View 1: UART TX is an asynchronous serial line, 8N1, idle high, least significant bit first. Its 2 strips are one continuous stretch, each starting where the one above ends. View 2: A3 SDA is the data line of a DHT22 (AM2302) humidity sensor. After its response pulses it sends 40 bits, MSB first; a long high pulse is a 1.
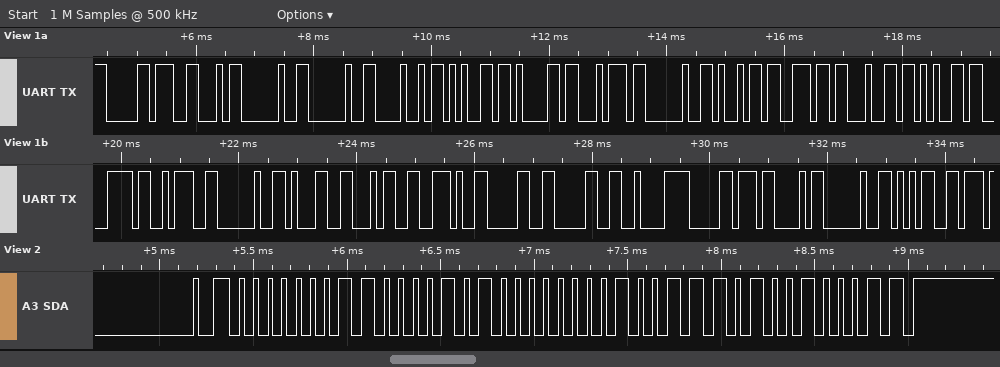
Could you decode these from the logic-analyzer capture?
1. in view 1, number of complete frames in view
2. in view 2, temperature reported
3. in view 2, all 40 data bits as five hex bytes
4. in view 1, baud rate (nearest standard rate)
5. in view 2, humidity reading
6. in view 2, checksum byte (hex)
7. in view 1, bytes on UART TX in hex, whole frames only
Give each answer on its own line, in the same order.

26
15.7 °C
01 85 00 9D 23
9600 baud
38.9 %
0x23
B0 46 20 20 48 65 61 74 20 69 6E 64 65 78 3A 20 31 34 2E 30 30 C2 B0 43 20 35
